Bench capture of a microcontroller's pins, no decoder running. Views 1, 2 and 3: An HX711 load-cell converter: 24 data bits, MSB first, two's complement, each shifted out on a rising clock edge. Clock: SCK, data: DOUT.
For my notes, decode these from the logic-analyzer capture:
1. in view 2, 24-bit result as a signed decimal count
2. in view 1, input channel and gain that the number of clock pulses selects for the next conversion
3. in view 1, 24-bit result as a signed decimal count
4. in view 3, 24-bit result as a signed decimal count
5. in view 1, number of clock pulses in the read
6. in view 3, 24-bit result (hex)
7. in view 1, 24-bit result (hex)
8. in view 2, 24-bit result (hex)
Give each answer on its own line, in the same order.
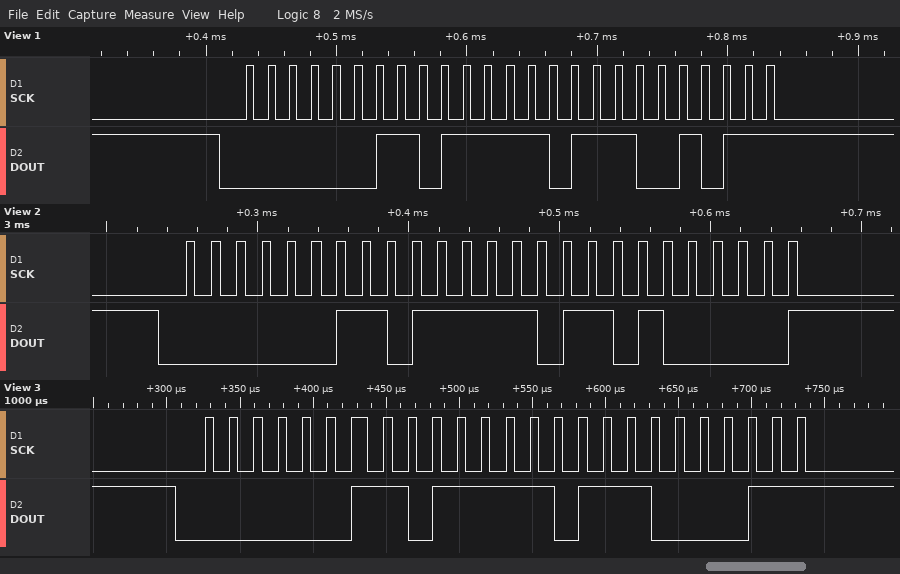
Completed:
228768
channel A, gain 128
228811
228803
25
0x037DC3
0x037DCB
0x037DA0
